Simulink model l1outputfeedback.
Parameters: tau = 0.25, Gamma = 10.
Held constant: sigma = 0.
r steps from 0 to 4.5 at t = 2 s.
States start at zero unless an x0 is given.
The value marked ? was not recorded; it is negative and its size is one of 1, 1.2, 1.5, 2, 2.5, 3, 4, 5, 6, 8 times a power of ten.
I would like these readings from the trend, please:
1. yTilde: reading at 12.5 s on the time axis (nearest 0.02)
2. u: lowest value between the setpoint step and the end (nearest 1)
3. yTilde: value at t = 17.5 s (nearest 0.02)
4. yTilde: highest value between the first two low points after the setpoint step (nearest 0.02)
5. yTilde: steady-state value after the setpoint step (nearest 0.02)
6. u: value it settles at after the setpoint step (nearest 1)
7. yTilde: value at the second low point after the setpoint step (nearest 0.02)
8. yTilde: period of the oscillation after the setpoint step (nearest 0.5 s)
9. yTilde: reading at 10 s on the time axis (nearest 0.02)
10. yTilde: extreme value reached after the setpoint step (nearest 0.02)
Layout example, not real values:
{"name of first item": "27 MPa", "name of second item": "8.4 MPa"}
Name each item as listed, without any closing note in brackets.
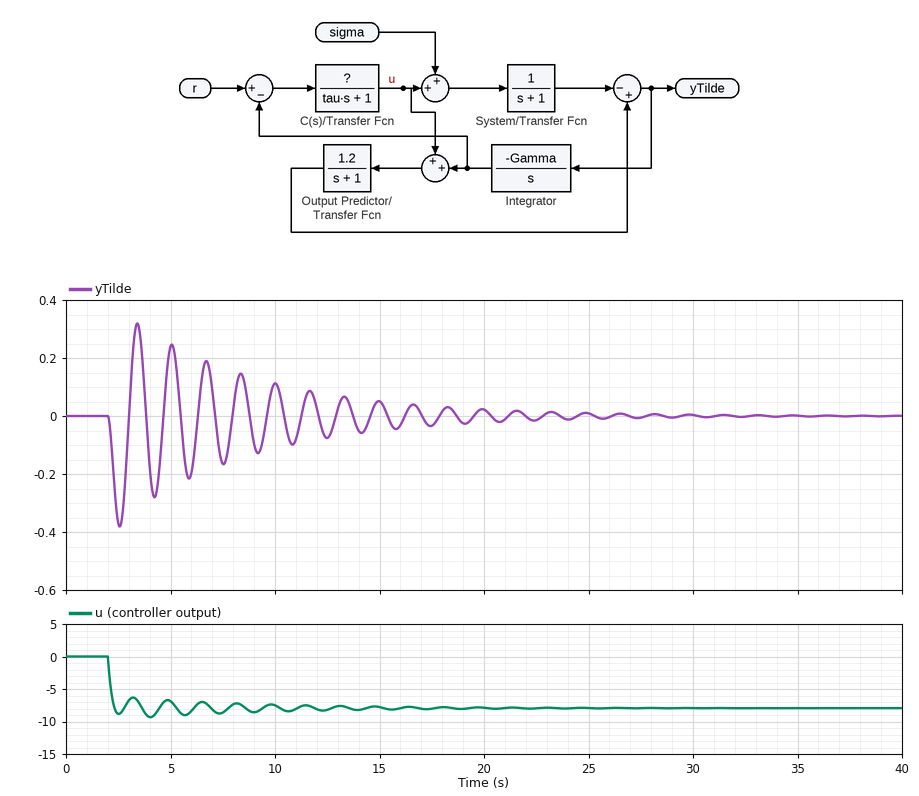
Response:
{"yTilde: reading at 12.5 s on the time axis": "-0.08", "u: lowest value between the setpoint step and the end": "-9", "yTilde: value at t = 17.5 s": "-0.04", "yTilde: highest value between the first two low points after the setpoint step": "0.32", "yTilde: steady-state value after the setpoint step": "0.00", "u: value it settles at after the setpoint step": "-8", "yTilde: value at the second low point after the setpoint step": "-0.28", "yTilde: period of the oscillation after the setpoint step": "1.5 s", "yTilde: reading at 10 s on the time axis": "0.12", "yTilde: extreme value reached after the setpoint step": "-0.38"}
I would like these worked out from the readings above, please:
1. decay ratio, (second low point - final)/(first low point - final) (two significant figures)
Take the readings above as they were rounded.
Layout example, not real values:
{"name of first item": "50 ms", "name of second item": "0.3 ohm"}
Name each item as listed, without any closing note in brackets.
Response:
{"decay ratio, (second low point - final)/(first low point - final)": "0.74"}
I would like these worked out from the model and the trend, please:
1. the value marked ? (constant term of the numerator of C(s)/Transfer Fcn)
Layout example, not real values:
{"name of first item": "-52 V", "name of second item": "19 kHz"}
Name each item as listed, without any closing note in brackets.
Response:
{"the value marked ? (constant term of the numerator of C(s)/Transfer Fcn)": "-2.5"}
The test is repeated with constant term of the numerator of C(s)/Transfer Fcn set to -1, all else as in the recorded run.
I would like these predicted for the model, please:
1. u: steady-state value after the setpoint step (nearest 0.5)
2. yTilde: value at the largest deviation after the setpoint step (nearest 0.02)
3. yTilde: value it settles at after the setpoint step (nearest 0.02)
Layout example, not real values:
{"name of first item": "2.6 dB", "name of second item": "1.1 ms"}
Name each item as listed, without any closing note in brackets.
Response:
{"u: steady-state value after the setpoint step": "-4.0", "yTilde: value at the largest deviation after the setpoint step": "-0.16", "yTilde: value it settles at after the setpoint step": "0.00"}
